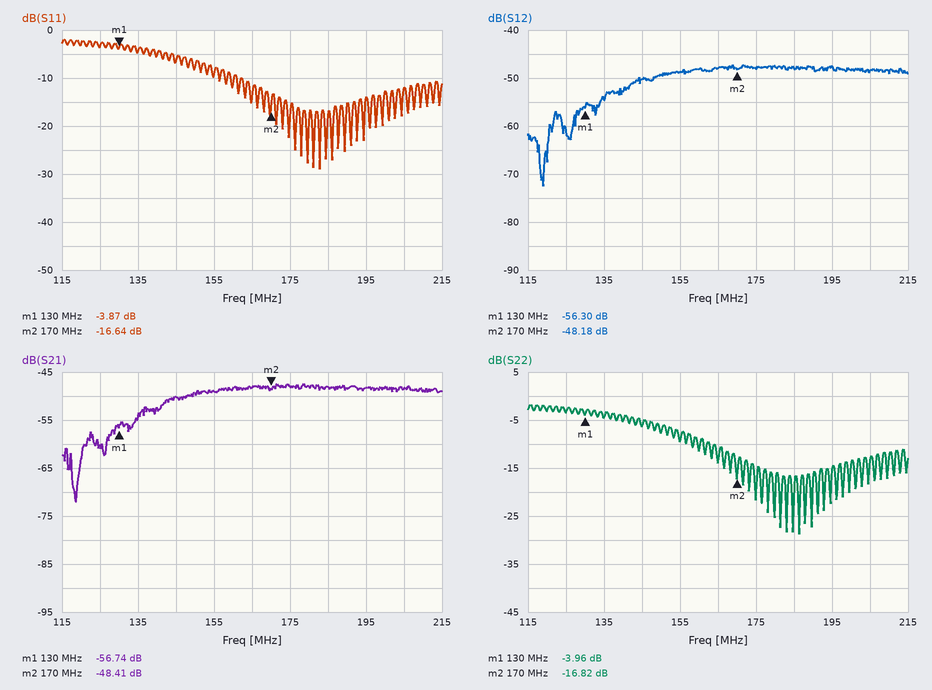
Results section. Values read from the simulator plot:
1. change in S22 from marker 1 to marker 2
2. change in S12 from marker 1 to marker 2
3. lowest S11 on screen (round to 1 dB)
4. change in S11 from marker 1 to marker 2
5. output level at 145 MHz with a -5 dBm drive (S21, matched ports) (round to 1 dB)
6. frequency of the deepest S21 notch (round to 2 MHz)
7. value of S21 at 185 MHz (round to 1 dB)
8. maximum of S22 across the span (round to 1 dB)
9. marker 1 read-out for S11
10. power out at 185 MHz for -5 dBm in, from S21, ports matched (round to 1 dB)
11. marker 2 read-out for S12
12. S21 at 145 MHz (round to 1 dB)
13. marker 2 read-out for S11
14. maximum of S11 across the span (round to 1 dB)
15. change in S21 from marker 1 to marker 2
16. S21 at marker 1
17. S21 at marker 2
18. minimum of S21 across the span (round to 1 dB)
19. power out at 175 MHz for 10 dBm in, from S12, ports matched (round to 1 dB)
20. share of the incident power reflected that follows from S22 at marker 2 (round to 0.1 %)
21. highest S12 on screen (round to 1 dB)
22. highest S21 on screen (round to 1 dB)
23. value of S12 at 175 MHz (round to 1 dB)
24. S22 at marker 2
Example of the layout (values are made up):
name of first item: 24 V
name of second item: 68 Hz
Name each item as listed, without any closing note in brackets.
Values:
change in S22 from marker 1 to marker 2: -12.86 dB
change in S12 from marker 1 to marker 2: 8.12 dB
lowest S11 on screen: -29 dB
change in S11 from marker 1 to marker 2: -12.77 dB
output level at 145 MHz with a -5 dBm drive (S21, matched ports): -55 dBm
frequency of the deepest S21 notch: 118 MHz
value of S21 at 185 MHz: -48 dB
maximum of S22 across the span: -2 dB
marker 1 read-out for S11: -3.87 dB
power out at 185 MHz for -5 dBm in, from S21, ports matched: -53 dBm
marker 2 read-out for S12: -48.18 dB
S21 at 145 MHz: -50 dB
marker 2 read-out for S11: -16.64 dB
maximum of S11 across the span: -2 dB
change in S21 from marker 1 to marker 2: 8.33 dB
S21 at marker 1: -56.74 dB
S21 at marker 2: -48.41 dB
minimum of S21 across the span: -72 dB
power out at 175 MHz for 10 dBm in, from S12, ports matched: -38 dBm
share of the incident power reflected that follows from S22 at marker 2: 2.1 %
highest S12 on screen: -47 dB
highest S21 on screen: -47 dB
value of S12 at 175 MHz: -48 dB
S22 at marker 2: -16.82 dB
